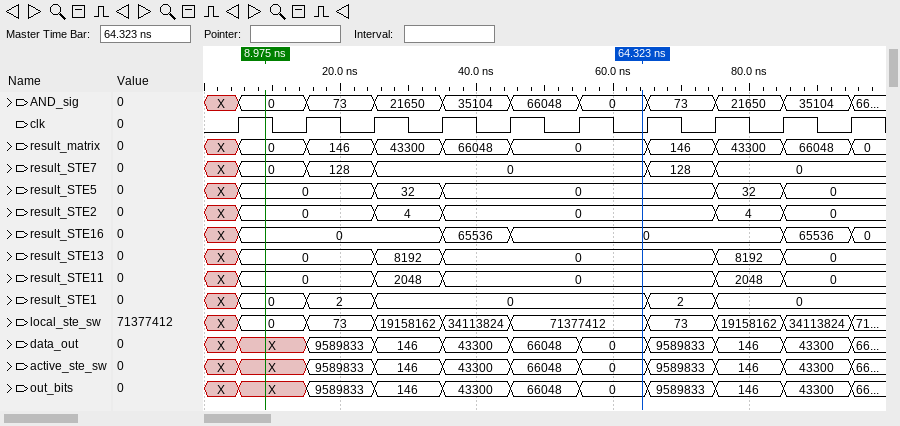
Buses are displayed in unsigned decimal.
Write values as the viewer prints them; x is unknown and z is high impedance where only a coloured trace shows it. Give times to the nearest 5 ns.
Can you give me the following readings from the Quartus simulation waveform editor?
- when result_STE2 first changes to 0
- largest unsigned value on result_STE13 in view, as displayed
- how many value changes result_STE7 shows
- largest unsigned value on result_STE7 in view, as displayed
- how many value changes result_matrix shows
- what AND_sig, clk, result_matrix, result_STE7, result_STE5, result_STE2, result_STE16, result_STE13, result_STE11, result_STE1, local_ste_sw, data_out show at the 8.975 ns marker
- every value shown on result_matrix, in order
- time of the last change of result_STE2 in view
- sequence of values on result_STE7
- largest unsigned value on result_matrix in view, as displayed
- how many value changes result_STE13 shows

5 ns
8192
5
128
9
AND_sig=0, clk=1, result_matrix=0, result_STE7=0, result_STE5=0, result_STE2=0, result_STE16=0, result_STE13=0, result_STE11=0, result_STE1=0, local_ste_sw=0, data_out=X
X, 0, 146, 43300, 66048, 0, 146, 43300, 66048, 0
85 ns
X, 0, 128, 0, 128, 0
66048
5
